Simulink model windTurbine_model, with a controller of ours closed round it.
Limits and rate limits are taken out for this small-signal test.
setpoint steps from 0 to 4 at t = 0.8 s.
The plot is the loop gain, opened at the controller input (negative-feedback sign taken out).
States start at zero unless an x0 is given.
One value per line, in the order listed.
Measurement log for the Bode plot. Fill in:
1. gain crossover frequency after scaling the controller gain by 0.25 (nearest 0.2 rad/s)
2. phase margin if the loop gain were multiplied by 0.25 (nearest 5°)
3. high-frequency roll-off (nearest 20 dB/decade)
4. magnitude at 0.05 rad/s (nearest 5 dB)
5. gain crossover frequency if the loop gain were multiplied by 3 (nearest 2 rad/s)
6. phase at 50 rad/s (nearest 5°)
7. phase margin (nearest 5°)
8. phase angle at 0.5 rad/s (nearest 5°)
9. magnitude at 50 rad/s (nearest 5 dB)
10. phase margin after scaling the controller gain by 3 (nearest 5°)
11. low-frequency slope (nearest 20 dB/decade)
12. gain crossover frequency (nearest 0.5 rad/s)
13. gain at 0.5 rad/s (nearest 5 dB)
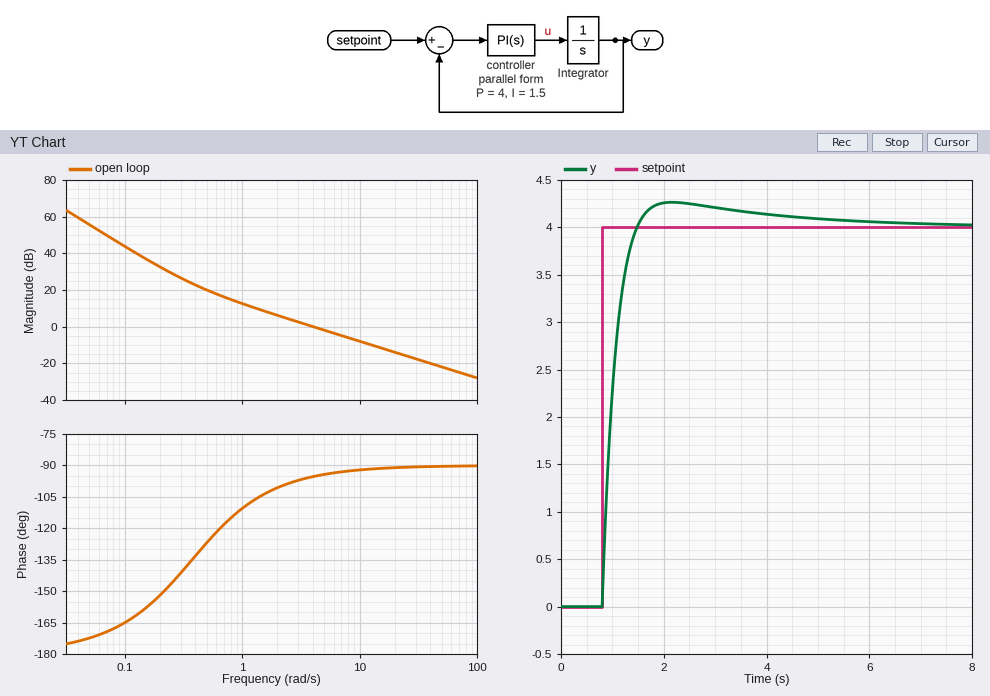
1.0 rad/s
70°
-20 dB/decade
55 dB
12 rad/s
-90°
85°
-125°
-20 dB
90°
-40 dB/decade
4.0 rad/s
20 dB
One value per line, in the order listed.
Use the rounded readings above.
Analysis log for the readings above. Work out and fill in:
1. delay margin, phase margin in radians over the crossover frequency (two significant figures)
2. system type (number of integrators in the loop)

0.37 s
2
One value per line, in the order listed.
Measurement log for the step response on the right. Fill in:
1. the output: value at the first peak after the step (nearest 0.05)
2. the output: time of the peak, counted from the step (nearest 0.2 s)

4.25
1.4 s
